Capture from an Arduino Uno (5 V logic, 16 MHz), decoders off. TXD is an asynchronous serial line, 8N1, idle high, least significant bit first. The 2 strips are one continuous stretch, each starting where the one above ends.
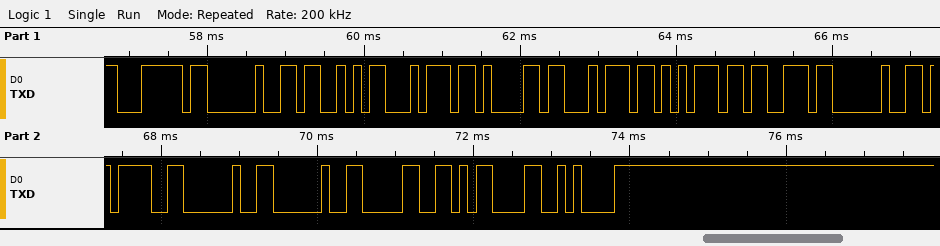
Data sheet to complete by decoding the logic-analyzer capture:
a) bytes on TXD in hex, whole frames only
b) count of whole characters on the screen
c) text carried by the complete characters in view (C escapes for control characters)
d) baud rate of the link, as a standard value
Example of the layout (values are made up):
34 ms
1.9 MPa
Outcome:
7C 20 53 74 61 74 75 73 20 3D 20 20 30 0D 0A
15
"| Status =  0\r\n"
9600 baud
